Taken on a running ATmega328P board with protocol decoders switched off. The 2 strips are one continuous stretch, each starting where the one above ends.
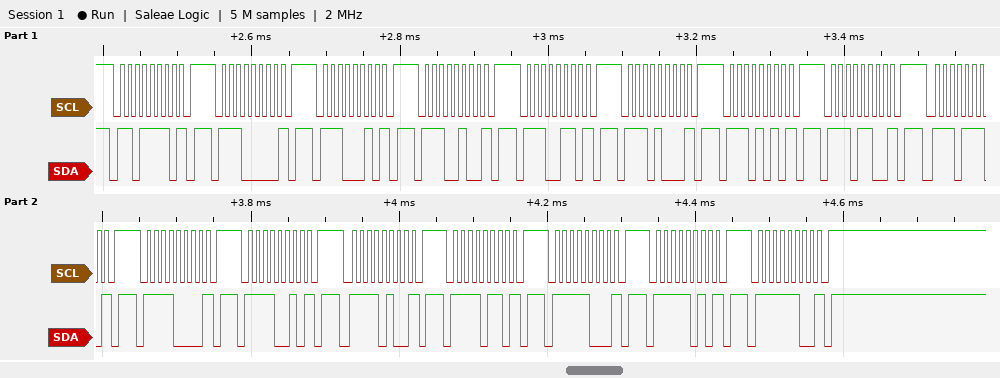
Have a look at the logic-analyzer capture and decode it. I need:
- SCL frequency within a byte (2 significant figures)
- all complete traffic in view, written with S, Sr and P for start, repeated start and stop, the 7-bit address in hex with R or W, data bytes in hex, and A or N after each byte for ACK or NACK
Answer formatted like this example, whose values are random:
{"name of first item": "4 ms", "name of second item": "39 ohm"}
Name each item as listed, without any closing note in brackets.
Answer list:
{"SCL frequency within a byte": "100 kHz", "all complete traffic in view, written with S, Sr and P for start, repeated start and stop, the 7-bit address in hex with R or W, data bytes in hex, and A or N after each byte for ACK or NACK": "S 6FW N P S 70W N P S 71W N P S 72W N P S 73W N P S 74W N P S 75W N P S 76W N P S 77W N P S 78W N P S 79W N P S 7AW N P S 7BW N P S 7CW N P S 7DW N P S 7EW N P"}
